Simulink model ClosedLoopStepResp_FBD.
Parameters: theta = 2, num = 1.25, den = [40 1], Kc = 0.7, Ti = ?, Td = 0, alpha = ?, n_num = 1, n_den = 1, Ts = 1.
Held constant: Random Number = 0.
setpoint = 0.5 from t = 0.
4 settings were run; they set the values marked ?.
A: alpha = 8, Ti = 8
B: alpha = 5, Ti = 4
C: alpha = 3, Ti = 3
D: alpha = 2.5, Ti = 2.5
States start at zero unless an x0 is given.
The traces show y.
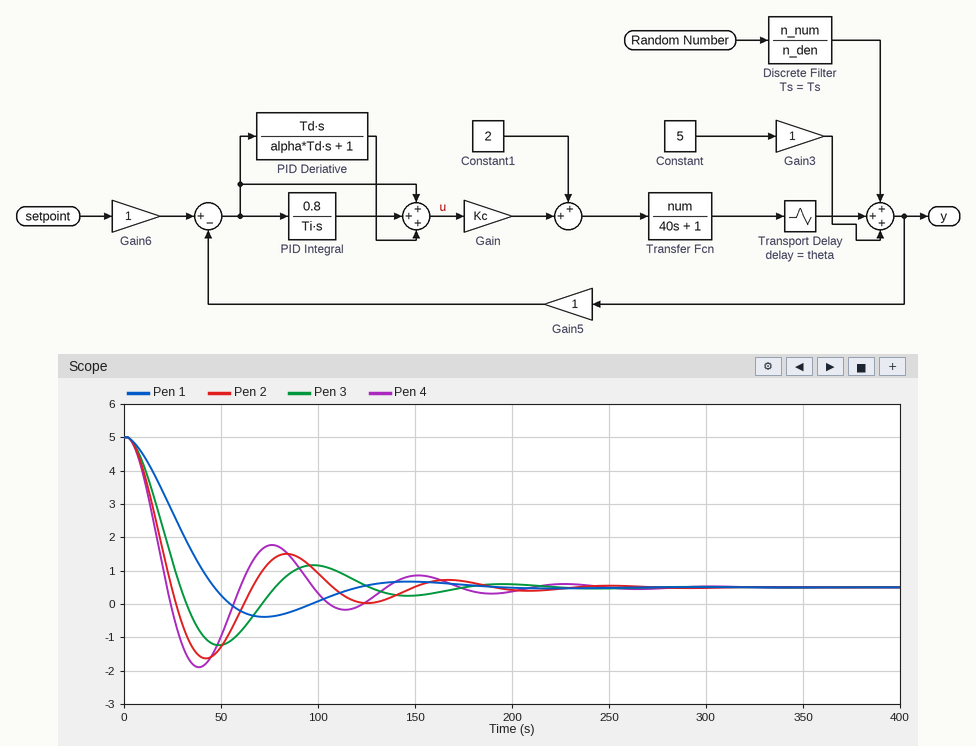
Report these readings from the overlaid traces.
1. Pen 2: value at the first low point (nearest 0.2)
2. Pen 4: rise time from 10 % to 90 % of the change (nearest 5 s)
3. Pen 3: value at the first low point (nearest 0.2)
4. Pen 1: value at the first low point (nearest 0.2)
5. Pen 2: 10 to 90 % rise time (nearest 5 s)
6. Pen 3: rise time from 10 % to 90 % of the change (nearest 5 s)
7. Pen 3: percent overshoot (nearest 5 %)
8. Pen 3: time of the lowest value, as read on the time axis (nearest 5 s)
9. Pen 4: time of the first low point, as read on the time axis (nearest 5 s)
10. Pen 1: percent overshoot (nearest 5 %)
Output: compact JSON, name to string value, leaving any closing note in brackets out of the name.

{"Pen 2: value at the first low point": "-1.6", "Pen 4: rise time from 10 % to 90 % of the change": "15 s", "Pen 3: value at the first low point": "-1.2", "Pen 1: value at the first low point": "-0.4", "Pen 2: 10 to 90 % rise time": "15 s", "Pen 3: rise time from 10 % to 90 % of the change": "20 s", "Pen 3: percent overshoot": "40 %", "Pen 3: time of the lowest value, as read on the time axis": "50 s", "Pen 4: time of the first low point, as read on the time axis": "40 s", "Pen 1: percent overshoot": "20 %"}
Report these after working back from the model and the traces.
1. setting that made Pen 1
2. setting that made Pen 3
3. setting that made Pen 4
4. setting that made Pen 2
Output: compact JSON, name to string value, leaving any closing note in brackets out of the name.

{"setting that made Pen 1": "A", "setting that made Pen 3": "B", "setting that made Pen 4": "D", "setting that made Pen 2": "C"}
